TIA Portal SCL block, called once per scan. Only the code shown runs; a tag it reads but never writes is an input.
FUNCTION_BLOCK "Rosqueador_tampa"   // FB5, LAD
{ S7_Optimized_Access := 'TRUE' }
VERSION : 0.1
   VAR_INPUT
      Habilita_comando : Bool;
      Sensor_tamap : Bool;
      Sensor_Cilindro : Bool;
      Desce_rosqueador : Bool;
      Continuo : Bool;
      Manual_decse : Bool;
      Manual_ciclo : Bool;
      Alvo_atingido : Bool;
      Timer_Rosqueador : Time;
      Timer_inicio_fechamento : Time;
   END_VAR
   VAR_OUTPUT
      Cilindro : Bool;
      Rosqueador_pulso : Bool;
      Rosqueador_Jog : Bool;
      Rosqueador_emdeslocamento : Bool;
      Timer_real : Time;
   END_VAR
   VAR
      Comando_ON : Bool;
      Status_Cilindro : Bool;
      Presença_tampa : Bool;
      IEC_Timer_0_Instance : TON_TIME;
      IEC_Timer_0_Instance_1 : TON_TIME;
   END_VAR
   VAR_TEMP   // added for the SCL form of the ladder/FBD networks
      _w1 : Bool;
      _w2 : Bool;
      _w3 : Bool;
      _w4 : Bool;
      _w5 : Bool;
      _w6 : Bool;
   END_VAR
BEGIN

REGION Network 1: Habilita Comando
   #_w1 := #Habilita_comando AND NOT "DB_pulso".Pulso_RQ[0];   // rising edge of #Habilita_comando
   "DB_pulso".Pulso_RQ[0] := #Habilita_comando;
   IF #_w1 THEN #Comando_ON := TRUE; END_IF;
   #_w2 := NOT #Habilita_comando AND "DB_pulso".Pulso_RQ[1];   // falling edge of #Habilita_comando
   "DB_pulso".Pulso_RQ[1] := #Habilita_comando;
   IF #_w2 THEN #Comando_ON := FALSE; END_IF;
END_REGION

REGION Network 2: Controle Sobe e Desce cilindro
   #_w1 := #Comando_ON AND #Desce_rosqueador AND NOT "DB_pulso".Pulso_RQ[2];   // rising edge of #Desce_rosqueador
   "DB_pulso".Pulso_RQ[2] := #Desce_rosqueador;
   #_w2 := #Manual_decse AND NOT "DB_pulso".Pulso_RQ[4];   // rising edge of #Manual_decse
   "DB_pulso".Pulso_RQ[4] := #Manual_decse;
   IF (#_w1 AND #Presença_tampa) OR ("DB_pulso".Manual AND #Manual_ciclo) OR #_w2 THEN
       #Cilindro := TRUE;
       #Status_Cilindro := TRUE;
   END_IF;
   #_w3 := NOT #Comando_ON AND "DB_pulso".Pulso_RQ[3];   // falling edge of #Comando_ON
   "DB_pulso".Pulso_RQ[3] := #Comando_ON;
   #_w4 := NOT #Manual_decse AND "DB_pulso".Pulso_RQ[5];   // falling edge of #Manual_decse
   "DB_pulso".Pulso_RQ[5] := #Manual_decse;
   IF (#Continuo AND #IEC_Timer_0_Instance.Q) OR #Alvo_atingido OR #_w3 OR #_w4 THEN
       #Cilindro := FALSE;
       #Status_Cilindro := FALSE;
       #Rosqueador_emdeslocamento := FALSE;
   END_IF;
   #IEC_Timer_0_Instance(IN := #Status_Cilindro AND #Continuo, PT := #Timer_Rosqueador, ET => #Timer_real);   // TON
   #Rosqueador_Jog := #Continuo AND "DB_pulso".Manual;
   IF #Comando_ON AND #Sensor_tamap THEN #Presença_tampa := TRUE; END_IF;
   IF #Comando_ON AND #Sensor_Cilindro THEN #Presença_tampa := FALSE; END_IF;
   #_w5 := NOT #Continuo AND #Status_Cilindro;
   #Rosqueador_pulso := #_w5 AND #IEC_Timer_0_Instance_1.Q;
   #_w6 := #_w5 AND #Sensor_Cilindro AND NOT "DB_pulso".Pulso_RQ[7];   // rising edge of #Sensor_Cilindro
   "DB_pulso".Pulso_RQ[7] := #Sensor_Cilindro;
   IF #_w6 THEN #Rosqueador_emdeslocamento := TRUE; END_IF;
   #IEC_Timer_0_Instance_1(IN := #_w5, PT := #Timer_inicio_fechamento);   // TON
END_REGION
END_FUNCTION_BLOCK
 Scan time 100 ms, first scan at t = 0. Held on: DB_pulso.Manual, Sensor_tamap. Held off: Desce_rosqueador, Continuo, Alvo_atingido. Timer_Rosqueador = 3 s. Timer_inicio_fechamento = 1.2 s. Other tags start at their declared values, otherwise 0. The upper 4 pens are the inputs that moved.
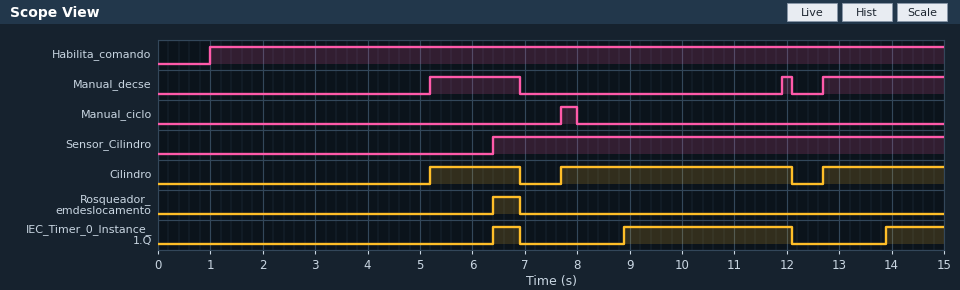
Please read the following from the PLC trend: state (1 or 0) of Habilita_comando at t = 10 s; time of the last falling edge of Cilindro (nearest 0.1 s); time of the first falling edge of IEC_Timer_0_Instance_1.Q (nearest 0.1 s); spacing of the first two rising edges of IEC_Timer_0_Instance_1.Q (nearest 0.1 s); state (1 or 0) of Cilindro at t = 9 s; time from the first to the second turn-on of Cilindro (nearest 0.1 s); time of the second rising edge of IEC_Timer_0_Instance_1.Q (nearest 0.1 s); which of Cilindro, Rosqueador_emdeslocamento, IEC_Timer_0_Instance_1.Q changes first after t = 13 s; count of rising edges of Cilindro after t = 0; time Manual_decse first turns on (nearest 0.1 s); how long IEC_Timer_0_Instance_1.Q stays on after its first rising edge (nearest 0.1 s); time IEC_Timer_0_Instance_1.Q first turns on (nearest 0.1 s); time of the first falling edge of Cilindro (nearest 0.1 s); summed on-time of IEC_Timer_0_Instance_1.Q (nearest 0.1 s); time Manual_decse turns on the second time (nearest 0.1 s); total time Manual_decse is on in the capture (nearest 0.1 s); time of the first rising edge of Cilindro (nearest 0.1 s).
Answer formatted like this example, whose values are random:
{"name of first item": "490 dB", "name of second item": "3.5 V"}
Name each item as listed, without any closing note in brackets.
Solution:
{"state (1 or 0) of Habilita_comando at t = 10 s": "1", "time of the last falling edge of Cilindro": "12.1 s", "time of the first falling edge of IEC_Timer_0_Instance_1.Q": "6.9 s", "spacing of the first two rising edges of IEC_Timer_0_Instance_1.Q": "2.5 s", "state (1 or 0) of Cilindro at t = 9 s": "1", "time from the first to the second turn-on of Cilindro": "2.5 s", "time of the second rising edge of IEC_Timer_0_Instance_1.Q": "8.9 s", "which of Cilindro, Rosqueador_emdeslocamento, IEC_Timer_0_Instance_1.Q changes first after t = 13 s": "IEC_Timer_0_Instance_1.Q", "count of rising edges of Cilindro after t = 0": "3", "time Manual_decse first turns on": "5.2 s", "how long IEC_Timer_0_Instance_1.Q stays on after its first rising edge": "0.5 s", "time IEC_Timer_0_Instance_1.Q first turns on": "6.4 s", "time of the first falling edge of Cilindro": "6.9 s", "summed on-time of IEC_Timer_0_Instance_1.Q": "4.8 s", "time Manual_decse turns on the second time": "11.9 s", "total time Manual_decse is on in the capture": "4.2 s", "time of the first rising edge of Cilindro": "5.2 s"}
